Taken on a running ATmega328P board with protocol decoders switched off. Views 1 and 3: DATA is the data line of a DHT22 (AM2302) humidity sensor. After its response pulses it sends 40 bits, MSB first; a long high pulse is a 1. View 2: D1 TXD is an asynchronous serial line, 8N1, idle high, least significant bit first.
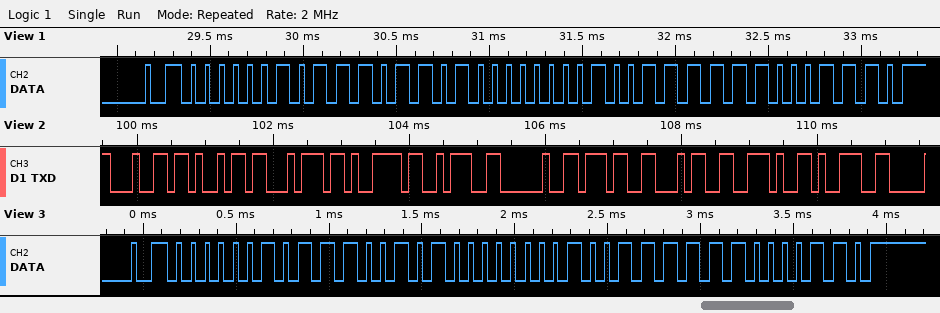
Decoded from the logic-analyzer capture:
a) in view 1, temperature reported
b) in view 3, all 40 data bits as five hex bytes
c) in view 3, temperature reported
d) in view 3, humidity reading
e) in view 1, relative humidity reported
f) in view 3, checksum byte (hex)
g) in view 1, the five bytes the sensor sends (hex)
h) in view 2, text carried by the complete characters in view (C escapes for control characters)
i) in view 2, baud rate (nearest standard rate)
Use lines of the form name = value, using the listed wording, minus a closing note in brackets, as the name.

in view 1, temperature reported = 15.9 °C
in view 3, all 40 data bits as five hex bytes = 02 E5 00 9F 86
in view 3, temperature reported = 15.9 °C
in view 3, humidity reading = 74.1 %
in view 1, relative humidity reported = 74.9 %
in view 3, checksum byte = 0x86
in view 1, the five bytes the sensor sends = 02 ED 00 9F 8E
in view 2, text carried by the complete characters in view = "dity: 74.9"
in view 2, baud rate = 9600 baud
